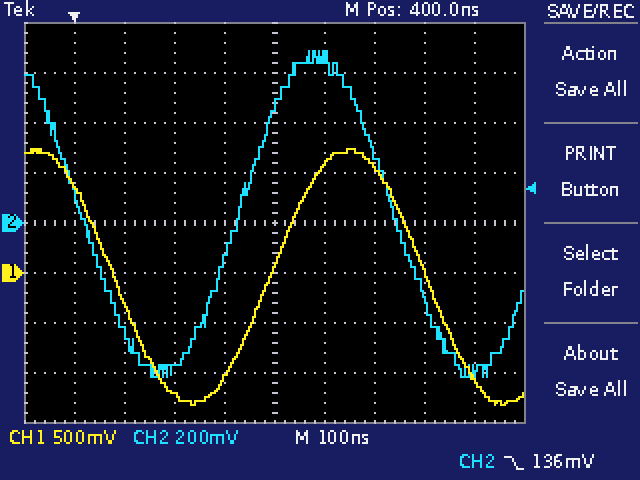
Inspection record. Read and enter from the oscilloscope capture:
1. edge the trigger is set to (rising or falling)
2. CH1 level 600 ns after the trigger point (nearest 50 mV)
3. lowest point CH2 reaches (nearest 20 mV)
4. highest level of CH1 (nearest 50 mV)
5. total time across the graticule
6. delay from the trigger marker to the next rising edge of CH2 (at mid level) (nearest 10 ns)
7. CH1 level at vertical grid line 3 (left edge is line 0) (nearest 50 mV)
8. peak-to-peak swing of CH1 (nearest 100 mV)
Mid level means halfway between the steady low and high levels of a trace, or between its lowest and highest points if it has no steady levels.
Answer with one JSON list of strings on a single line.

["falling", "1.05 V", "-620 mV", "1.25 V", "1 µs", "330 ns", "-1.20 V", "2.60 V"]
